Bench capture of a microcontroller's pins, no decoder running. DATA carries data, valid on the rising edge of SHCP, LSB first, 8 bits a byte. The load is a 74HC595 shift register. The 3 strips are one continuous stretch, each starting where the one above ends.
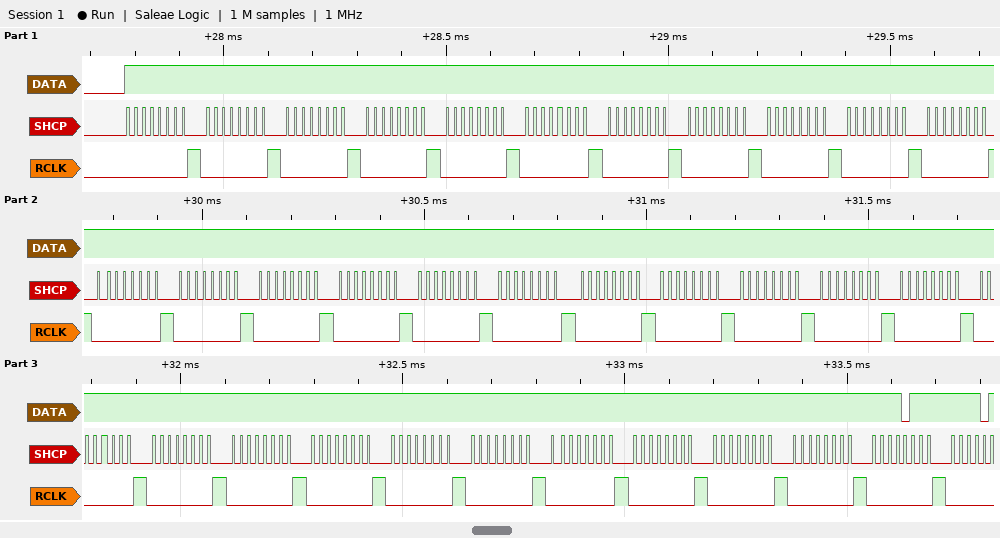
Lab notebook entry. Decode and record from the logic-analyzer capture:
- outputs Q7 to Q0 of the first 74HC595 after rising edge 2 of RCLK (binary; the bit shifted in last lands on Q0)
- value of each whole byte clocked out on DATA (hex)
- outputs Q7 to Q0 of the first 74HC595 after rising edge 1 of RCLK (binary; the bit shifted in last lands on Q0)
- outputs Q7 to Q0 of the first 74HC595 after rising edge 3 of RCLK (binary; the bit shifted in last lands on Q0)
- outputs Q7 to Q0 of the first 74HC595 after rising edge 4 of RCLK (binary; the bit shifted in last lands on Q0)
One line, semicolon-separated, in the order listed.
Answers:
11111111; FF FF FF FF FF FF FF FF FF FF FF FF FF FF FF FF FF FF FF FF FF FF FF FF FF FF FF FF FF FF FF FF EF; 11111111; 11111111; 11111111
